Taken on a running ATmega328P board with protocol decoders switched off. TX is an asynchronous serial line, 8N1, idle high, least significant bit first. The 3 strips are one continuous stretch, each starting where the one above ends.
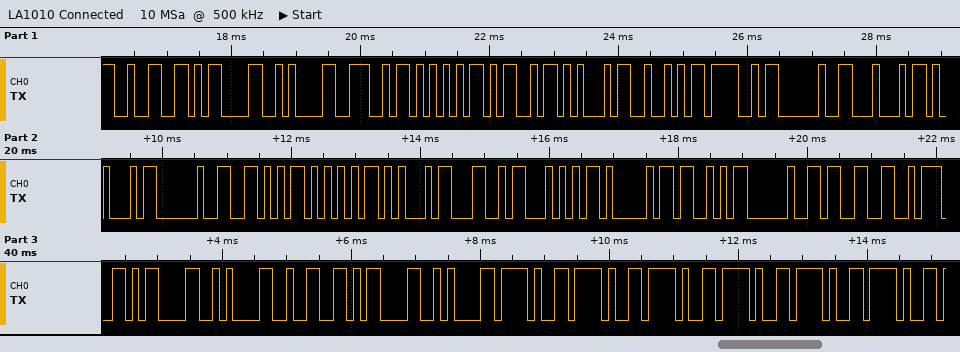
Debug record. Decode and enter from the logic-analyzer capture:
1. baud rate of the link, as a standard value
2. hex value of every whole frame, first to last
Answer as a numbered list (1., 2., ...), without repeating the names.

1. 9600 baud
2. 32 0D 0A 4E 55 4D 45 52 4F 20 44 45 20 56 55 45 4C 54 41 53 20 33 3A 0D 0A 32 0D 0A 2F 2F 2F 2F 2F 2F
